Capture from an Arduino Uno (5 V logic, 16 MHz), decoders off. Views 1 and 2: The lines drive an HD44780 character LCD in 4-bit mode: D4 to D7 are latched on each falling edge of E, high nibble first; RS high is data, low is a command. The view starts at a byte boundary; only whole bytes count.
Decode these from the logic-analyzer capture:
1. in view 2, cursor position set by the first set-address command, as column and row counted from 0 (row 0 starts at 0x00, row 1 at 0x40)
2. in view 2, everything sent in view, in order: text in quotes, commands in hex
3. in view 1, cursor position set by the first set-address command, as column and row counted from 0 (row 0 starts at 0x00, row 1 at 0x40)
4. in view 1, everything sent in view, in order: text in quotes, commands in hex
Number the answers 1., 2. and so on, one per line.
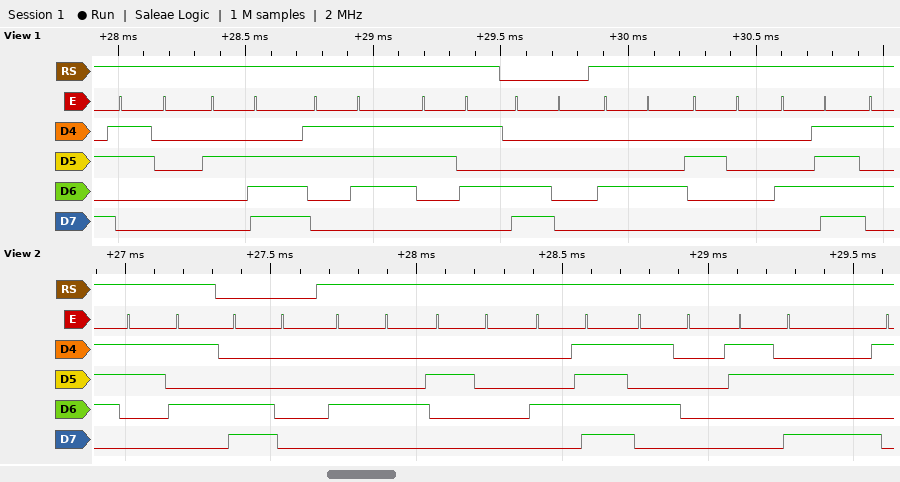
1. column 0, row 1
2. "5" 0xC0 "D OP:"
3. column 0, row 1
4. "0.75" 0xC0 "D O"
